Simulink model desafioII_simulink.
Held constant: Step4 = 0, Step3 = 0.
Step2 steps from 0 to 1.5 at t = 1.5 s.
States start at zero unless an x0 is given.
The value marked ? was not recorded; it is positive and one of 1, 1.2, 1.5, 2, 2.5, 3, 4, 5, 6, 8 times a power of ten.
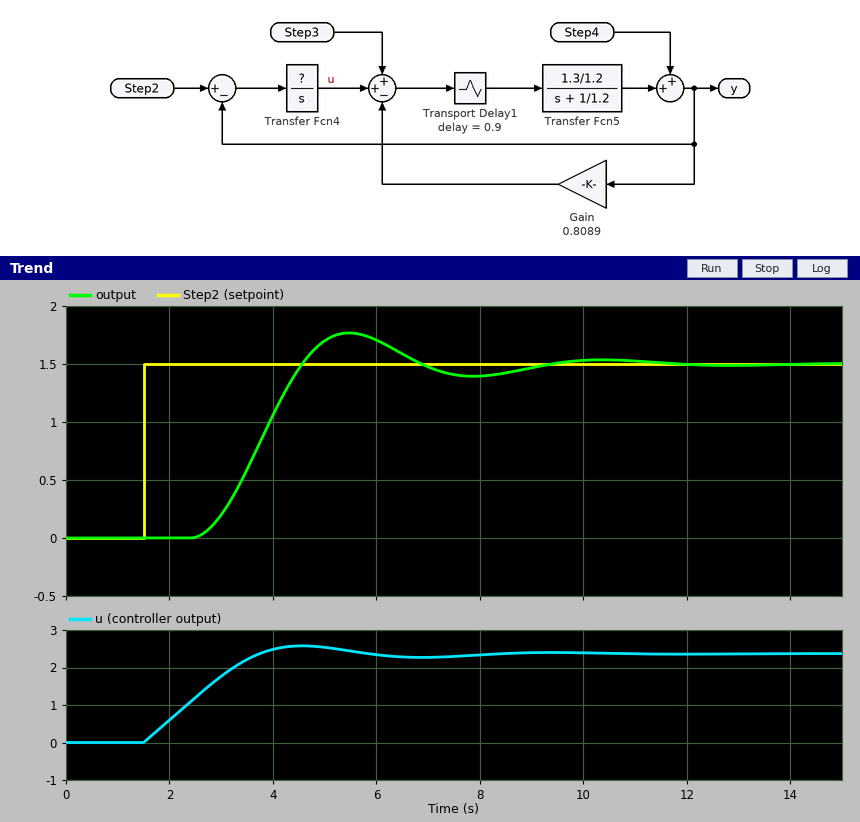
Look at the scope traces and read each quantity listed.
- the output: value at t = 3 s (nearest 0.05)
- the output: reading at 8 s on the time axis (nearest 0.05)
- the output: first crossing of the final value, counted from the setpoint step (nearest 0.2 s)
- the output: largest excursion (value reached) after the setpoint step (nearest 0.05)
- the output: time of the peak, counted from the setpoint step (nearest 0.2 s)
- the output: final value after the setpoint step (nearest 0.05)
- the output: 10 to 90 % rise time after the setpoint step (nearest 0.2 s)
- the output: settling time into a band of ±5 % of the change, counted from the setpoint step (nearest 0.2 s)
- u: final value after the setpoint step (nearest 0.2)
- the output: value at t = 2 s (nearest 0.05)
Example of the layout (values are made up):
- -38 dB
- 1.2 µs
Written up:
- 0.20
- 1.40
- 3.0 s
- 1.75
- 4.0 s
- 1.50
- 1.4 s
- 7.0 s
- 2.4
- 0.00
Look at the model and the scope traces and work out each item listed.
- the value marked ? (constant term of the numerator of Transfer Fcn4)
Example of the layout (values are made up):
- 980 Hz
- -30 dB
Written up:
- 0.8
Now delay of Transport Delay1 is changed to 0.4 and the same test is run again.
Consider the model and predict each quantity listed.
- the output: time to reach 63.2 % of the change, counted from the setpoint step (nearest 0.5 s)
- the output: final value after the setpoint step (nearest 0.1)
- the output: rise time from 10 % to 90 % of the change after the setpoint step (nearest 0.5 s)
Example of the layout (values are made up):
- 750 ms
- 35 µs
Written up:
- 2.0 s
- 1.5
- 2.5 s
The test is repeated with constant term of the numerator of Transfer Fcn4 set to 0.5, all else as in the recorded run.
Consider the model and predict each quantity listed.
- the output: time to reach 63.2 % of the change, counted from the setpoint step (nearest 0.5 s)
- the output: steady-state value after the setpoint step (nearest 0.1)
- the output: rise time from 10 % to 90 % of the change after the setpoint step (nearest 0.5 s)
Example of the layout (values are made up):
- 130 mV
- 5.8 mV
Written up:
- 3.0 s
- 1.5
- 4.0 s
